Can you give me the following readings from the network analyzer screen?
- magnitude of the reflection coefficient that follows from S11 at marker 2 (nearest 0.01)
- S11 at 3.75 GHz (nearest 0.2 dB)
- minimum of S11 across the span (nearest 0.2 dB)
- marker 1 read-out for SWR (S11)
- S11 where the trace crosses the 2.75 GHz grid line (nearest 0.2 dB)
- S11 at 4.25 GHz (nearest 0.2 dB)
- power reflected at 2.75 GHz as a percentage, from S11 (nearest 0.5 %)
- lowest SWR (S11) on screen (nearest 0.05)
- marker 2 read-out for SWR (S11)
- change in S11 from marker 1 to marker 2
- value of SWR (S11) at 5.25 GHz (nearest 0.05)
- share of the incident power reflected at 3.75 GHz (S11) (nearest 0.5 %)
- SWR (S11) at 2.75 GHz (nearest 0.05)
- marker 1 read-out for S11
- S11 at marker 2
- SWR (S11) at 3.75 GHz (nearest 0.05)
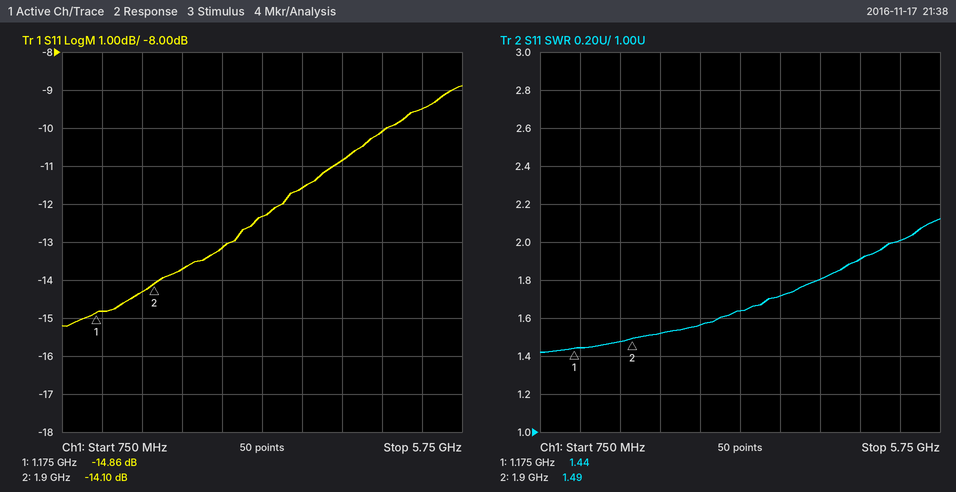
0.20
-11.6 dB
-15.2 dB
1.44
-13.2 dB
-10.8 dB
5.0 %
1.40
1.49
0.76 dB
2.00
7.0 %
1.55
-14.86 dB
-14.10 dB
1.70
